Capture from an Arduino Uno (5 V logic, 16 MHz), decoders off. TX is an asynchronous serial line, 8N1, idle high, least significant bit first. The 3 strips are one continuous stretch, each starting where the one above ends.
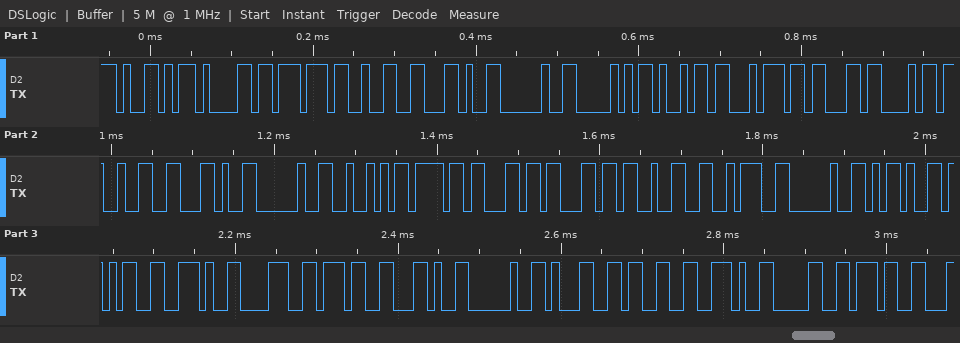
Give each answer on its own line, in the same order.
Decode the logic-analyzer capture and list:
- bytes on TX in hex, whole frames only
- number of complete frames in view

0x59 0x61 0x77 0x32 0x2C 0x20 0x50 0x69 0x74 0x63 0x68 0x32 0x2C 0x20 0x52 0x6F 0x6C 0x6C 0x32 0x3A 0x20 0x2D 0x35 0x2E 0x38 0x37 0x2C 0x20 0x31 0x33 0x2E 0x30 0x37
33
